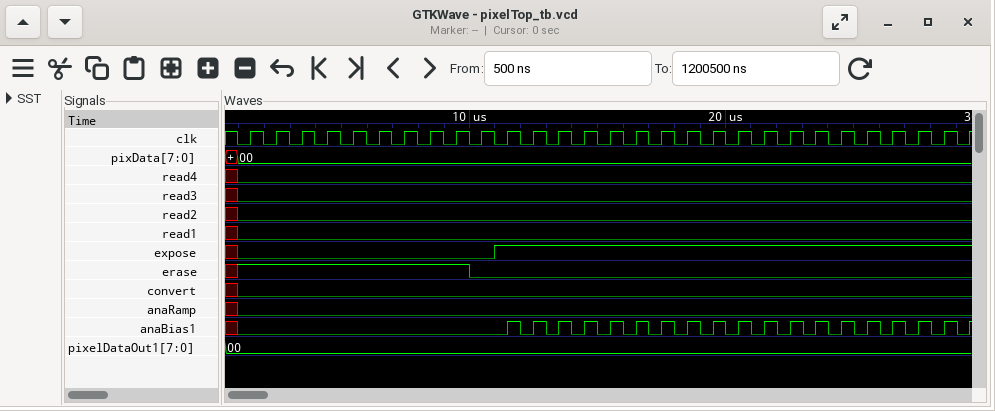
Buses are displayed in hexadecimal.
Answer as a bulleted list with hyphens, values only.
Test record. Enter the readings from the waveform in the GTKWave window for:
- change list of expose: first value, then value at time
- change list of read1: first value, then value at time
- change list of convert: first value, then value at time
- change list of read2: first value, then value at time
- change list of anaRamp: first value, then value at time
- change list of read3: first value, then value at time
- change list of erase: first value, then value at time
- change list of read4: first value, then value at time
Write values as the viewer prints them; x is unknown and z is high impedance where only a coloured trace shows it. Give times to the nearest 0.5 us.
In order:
- x, 0 at 1 us, 1 at 11 us
- x, 0 at 1 us
- x, 0 at 1 us
- x, 0 at 1 us
- x, 0 at 1 us
- x, 0 at 1 us
- x, 1 at 1 us, 0 at 10 us
- x, 0 at 1 us
